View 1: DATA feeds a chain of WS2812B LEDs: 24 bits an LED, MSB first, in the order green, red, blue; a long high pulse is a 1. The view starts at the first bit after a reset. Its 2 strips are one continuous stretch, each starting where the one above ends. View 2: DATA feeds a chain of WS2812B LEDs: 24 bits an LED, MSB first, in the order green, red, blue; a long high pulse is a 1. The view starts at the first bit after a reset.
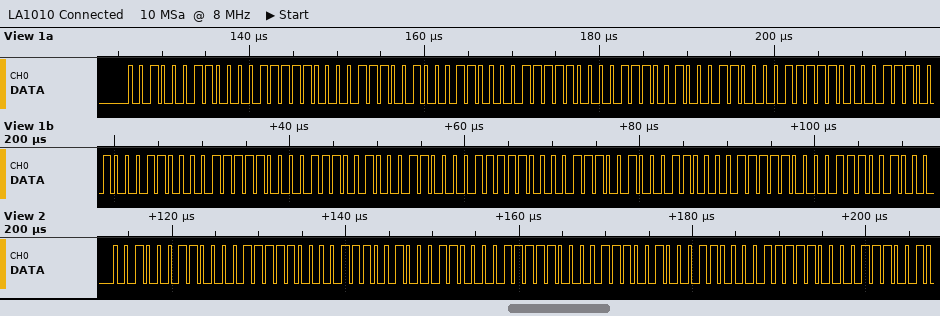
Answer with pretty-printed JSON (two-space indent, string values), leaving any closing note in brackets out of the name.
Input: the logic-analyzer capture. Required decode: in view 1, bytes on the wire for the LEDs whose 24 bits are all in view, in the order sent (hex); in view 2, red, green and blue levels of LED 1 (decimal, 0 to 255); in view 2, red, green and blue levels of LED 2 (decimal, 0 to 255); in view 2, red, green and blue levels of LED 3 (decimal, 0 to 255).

{
  "in view 1, bytes on the wire for the LEDs whose 24 bits are all in view, in the order sent": "23 0F 87 23 0F 87 23 0F 87 23 0F 87 23 0F 87 23 0F 87",
  "in view 2, red, green and blue levels of LED 1": "15, 35, 135",
  "in view 2, red, green and blue levels of LED 2": "15, 35, 135",
  "in view 2, red, green and blue levels of LED 3": "15, 35, 135"
}
